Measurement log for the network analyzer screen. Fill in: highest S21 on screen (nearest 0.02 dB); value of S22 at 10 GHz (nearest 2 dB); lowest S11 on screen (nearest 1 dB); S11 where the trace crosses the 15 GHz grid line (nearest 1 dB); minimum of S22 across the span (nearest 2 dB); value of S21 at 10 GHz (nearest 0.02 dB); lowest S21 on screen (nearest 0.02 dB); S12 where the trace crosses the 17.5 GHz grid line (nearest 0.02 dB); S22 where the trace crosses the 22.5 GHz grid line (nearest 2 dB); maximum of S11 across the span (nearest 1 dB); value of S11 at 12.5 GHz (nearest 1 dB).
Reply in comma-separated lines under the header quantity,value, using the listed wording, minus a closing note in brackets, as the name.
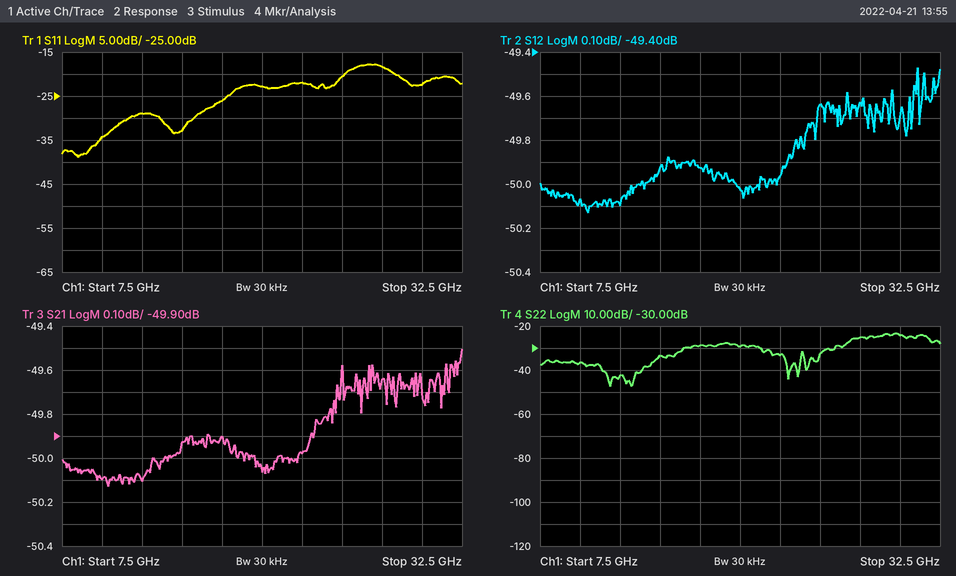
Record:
quantity,value
highest S21 on screen,-49.50 dB
value of S22 at 10 GHz,-36 dB
lowest S11 on screen,-39 dB
S11 where the trace crosses the 15 GHz grid line,-33 dB
minimum of S22 across the span,-48 dB
value of S21 at 10 GHz,-50.10 dB
lowest S21 on screen,-50.12 dB
S12 where the trace crosses the 17.5 GHz grid line,-49.92 dB
S22 where the trace crosses the 22.5 GHz grid line,-34 dB
maximum of S11 across the span,-18 dB
value of S11 at 12.5 GHz,-29 dB
